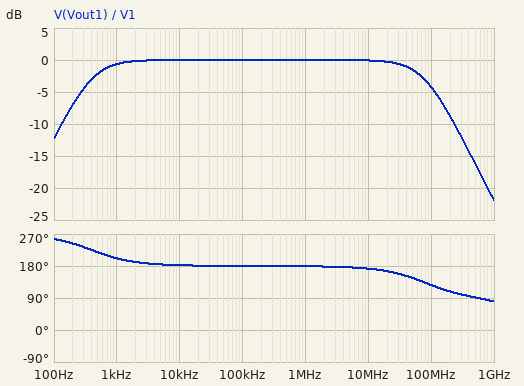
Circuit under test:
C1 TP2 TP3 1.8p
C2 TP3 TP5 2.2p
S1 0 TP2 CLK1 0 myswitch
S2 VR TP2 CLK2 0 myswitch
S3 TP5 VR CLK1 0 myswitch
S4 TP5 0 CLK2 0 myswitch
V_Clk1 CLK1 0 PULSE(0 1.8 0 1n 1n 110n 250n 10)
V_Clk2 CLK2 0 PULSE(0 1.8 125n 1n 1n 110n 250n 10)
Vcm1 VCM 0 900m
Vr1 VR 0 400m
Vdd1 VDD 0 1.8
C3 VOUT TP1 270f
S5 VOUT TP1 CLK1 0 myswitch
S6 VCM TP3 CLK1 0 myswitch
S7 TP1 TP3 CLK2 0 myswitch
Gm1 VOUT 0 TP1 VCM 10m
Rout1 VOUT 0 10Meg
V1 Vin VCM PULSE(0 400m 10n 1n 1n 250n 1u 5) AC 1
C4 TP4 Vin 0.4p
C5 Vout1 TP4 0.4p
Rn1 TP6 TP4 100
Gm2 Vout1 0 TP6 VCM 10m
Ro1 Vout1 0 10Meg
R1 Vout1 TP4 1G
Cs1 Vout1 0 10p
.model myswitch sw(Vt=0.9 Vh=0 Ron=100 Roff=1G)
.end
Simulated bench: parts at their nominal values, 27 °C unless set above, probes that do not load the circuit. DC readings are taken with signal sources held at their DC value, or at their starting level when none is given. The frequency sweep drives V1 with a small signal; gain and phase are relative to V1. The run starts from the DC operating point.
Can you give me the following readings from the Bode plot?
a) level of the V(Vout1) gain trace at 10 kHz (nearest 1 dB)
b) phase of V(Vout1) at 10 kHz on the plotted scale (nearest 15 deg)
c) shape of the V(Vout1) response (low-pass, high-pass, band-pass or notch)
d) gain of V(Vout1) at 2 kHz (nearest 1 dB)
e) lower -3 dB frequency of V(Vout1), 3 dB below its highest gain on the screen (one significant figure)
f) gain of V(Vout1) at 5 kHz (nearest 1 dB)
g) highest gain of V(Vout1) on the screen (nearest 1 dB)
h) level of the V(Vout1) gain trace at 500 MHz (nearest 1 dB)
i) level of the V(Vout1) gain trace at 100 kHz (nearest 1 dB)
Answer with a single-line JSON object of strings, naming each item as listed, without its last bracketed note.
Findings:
{"level of the V(Vout1) gain trace at 10 kHz": "0 dB", "phase of V(Vout1) at 10 kHz on the plotted scale": "180 deg", "shape of the V(Vout1) response": "band-pass", "gain of V(Vout1) at 2 kHz": "0 dB", "lower -3 dB frequency of V(Vout1), 3 dB below its highest gain on the screen": "400 Hz", "gain of V(Vout1) at 5 kHz": "0 dB", "highest gain of V(Vout1) on the screen": "0 dB", "level of the V(Vout1) gain trace at 500 MHz": "-16 dB", "level of the V(Vout1) gain trace at 100 kHz": "0 dB"}
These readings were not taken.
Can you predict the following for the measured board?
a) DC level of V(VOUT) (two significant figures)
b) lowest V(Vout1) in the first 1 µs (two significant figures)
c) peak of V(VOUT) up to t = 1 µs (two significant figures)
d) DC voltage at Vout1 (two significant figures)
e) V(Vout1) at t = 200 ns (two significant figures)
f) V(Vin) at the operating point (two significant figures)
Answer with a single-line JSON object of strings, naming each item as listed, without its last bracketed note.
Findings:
{"DC level of V(VOUT)": "900 mV", "lowest V(Vout1) in the first 1 µs": "500 mV", "peak of V(VOUT) up to t = 1 µs": "1.5 V", "DC voltage at Vout1": "900 mV", "V(Vout1) at t = 200 ns": "500 mV", "V(Vin) at the operating point": "900 mV"}
